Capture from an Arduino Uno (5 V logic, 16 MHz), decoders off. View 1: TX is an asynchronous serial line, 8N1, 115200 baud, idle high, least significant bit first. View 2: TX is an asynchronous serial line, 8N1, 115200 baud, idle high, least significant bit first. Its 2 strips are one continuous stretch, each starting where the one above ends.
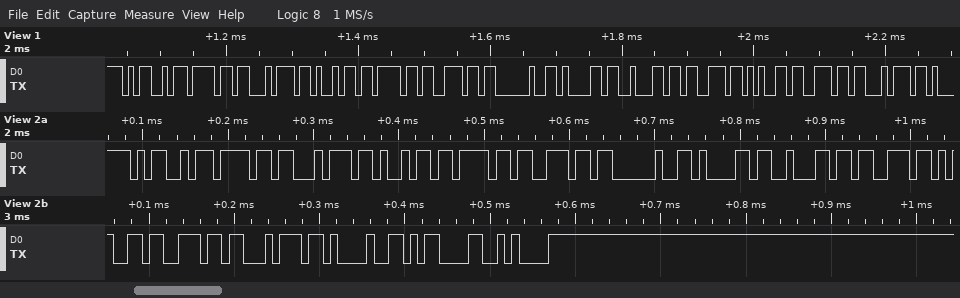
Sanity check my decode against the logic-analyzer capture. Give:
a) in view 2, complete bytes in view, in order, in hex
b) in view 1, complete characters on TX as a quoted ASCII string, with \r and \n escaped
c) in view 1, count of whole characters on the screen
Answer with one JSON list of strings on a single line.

["4D 6F 74 69 6F 6E 20 61 62 73 65 6E 74 21 0D 0A", "\"Motion absent\"", "13"]
